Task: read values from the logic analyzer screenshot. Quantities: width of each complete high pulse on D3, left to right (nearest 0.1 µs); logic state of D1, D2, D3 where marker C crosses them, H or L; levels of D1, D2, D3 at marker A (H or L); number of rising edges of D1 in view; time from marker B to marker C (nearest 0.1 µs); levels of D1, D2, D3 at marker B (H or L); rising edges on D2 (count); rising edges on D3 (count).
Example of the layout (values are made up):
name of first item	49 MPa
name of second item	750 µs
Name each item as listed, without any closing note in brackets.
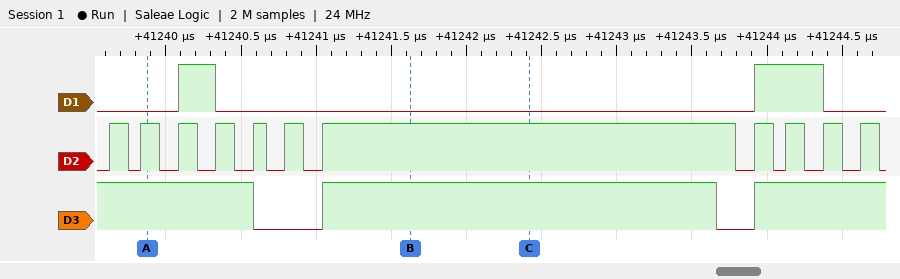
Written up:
width of each complete high pulse on D3, left to right	2.6 µs
logic state of D1, D2, D3 where marker C crosses them, H or L	D1=L, D2=H, D3=H
levels of D1, D2, D3 at marker A	D1=L, D2=H, D3=H
number of rising edges of D1 in view	2
time from marker B to marker C	0.8 µs
levels of D1, D2, D3 at marker B	D1=L, D2=H, D3=H
rising edges on D2	11
rising edges on D3	2
